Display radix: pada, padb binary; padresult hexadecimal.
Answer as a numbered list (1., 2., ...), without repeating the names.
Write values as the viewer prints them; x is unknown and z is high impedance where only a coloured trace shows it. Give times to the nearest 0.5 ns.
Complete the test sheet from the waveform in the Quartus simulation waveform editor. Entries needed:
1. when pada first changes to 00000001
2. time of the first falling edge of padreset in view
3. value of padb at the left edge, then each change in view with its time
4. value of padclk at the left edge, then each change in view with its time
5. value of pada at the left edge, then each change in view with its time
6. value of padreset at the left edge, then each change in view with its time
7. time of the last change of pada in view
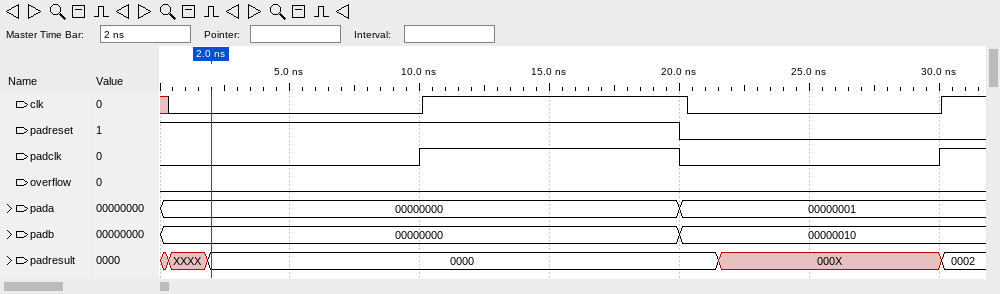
1. 20 ns
2. 20 ns
3. 00000000, 00000010 at 20 ns
4. 0, 1 at 10 ns, 0 at 20 ns, 1 at 30 ns
5. 00000000, 00000001 at 20 ns
6. 1, 0 at 20 ns
7. 20 ns
